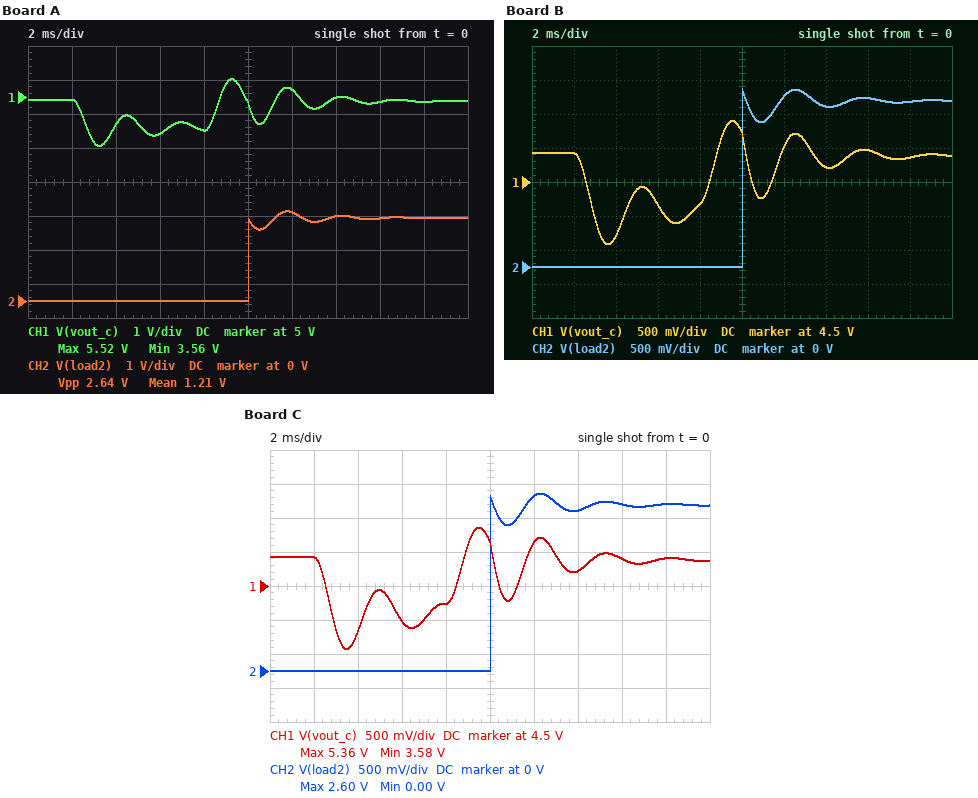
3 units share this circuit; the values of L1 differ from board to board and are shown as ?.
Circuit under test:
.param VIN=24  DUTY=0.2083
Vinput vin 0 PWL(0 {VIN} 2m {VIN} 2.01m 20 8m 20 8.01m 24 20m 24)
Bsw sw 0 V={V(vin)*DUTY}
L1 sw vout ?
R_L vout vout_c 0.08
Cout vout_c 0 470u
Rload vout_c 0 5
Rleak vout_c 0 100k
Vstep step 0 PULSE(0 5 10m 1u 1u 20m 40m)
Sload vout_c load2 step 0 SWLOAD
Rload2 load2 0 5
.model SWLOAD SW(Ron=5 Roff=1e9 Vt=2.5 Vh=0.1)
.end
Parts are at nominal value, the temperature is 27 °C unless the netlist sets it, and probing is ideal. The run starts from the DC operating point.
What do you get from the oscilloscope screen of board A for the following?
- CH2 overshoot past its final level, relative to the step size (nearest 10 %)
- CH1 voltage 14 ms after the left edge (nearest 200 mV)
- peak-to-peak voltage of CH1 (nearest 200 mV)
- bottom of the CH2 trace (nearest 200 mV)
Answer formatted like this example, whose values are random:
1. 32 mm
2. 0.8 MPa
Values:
1. 10 %
2. 5.0 V
3. 2.0 V
4. 0 V
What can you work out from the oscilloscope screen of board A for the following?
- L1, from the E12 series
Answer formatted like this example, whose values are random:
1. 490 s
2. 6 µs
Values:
1. 330 µH
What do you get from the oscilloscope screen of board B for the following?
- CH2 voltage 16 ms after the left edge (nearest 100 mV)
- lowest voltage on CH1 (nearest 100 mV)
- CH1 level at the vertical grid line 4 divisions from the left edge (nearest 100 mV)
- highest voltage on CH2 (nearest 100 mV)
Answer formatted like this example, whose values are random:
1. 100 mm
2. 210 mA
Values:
1. 2.5 V
2. 3.6 V
3. 4.2 V
4. 2.6 V
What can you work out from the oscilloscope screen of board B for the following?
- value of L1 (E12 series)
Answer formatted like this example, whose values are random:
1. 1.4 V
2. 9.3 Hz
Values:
1. 560 µH
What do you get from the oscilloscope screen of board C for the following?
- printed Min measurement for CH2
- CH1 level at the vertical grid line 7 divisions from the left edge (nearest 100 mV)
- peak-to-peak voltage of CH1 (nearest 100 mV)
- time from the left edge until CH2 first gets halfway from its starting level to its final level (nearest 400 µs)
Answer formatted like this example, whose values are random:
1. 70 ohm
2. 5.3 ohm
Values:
1. 0.00 V
2. 4.7 V
3. 1.8 V
4. 10.0 ms
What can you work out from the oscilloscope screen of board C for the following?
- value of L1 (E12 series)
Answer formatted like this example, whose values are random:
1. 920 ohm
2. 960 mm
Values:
1. 470 µH
